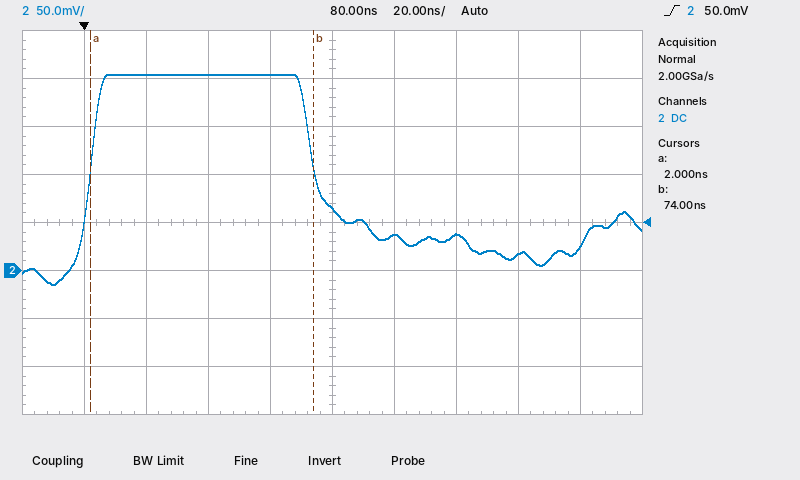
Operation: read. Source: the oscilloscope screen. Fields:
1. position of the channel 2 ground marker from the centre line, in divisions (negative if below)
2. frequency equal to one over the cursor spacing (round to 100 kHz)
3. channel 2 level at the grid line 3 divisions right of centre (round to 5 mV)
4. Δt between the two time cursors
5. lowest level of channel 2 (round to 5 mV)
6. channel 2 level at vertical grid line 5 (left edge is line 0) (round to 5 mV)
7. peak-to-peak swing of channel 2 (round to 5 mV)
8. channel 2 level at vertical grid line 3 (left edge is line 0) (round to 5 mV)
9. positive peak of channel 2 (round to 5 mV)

-1.0 div
13.9 MHz
15 mV
72 ns
-15 mV
65 mV
220 mV
205 mV
205 mV
